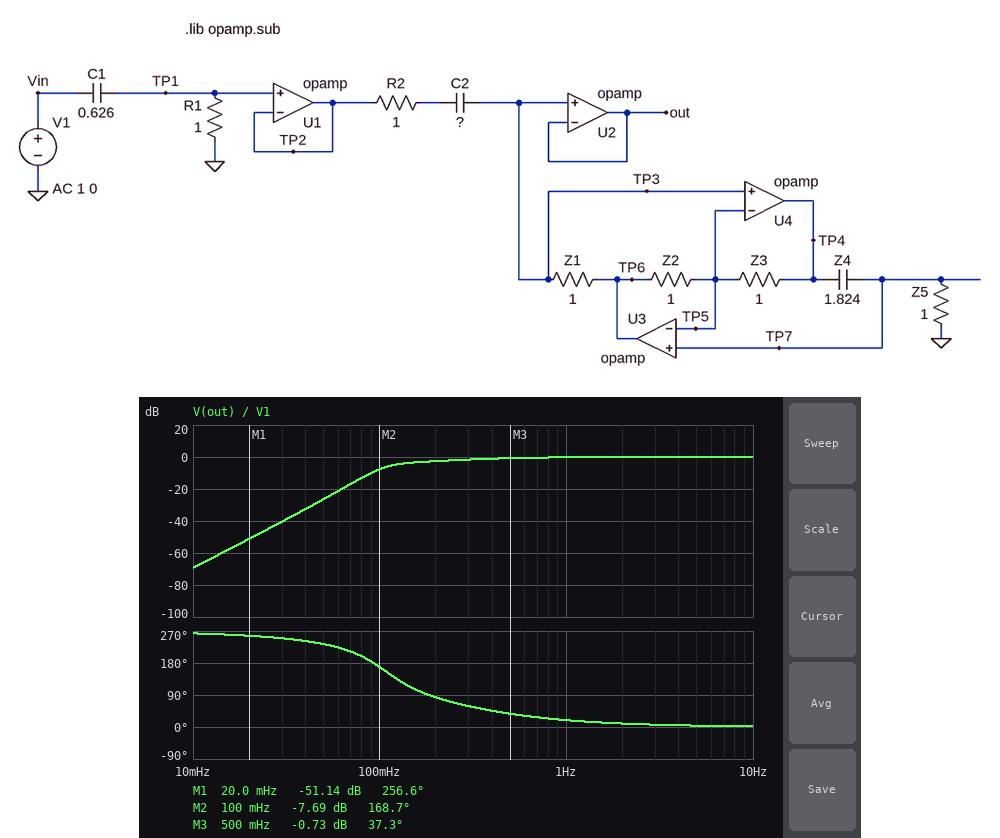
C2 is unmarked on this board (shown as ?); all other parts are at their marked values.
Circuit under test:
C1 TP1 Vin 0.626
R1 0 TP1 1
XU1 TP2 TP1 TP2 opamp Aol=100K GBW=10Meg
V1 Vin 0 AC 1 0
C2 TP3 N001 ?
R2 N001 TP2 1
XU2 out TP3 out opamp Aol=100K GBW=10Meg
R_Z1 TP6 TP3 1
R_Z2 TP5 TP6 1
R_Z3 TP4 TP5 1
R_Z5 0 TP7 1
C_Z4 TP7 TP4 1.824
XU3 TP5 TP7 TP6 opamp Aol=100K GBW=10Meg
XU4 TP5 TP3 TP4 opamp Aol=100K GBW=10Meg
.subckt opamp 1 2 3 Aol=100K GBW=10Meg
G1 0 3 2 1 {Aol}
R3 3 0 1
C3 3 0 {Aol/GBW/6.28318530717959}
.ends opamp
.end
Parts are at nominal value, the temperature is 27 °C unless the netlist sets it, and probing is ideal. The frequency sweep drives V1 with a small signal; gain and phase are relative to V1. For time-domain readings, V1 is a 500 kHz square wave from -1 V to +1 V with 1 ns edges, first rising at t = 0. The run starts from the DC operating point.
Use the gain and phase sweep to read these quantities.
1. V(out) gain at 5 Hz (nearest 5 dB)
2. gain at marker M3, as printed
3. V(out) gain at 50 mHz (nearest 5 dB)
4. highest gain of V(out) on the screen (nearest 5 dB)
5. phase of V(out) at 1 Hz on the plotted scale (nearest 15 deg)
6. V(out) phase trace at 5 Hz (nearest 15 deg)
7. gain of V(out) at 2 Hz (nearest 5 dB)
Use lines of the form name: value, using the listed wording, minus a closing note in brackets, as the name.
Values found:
V(out) gain at 5 Hz: 0 dB
gain at marker M3, as printed: -0.73 dB
V(out) gain at 50 mHz: -25 dB
highest gain of V(out) on the screen: 0 dB
phase of V(out) at 1 Hz on the plotted scale: 15 deg
V(out) phase trace at 5 Hz: 0 deg
gain of V(out) at 2 Hz: 0 dB
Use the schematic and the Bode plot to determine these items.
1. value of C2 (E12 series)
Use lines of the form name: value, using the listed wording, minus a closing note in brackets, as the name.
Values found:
value of C2: 1.2 F
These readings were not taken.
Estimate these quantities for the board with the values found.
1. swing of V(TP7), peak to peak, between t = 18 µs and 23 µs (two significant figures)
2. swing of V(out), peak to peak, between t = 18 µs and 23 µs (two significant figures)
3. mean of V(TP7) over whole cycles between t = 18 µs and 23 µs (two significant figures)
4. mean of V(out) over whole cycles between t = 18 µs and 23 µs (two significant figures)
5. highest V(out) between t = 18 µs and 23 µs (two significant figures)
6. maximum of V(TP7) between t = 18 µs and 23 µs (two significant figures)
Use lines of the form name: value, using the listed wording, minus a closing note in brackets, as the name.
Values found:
swing of V(TP7), peak to peak, between t = 18 µs and 23 µs: 2.0 V
swing of V(out), peak to peak, between t = 18 µs and 23 µs: 2.0 V
mean of V(TP7) over whole cycles between t = 18 µs and 23 µs: 1.0 V
mean of V(out) over whole cycles between t = 18 µs and 23 µs: 1.0 V
highest V(out) between t = 18 µs and 23 µs: 2.0 V
maximum of V(TP7) between t = 18 µs and 23 µs: 2.0 V
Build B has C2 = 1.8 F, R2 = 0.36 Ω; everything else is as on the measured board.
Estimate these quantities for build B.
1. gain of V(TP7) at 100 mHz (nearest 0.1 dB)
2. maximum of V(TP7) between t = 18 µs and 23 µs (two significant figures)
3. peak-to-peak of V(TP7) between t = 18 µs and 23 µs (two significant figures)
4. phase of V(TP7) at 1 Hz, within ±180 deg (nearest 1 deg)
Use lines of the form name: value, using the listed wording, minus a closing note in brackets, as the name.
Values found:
gain of V(TP7) at 100 mHz: -0.5 dB
maximum of V(TP7) between t = 18 µs and 23 µs: 2.1 V
peak-to-peak of V(TP7) between t = 18 µs and 23 µs: 2.2 V
phase of V(TP7) at 1 Hz, within ±180 deg: 16 deg
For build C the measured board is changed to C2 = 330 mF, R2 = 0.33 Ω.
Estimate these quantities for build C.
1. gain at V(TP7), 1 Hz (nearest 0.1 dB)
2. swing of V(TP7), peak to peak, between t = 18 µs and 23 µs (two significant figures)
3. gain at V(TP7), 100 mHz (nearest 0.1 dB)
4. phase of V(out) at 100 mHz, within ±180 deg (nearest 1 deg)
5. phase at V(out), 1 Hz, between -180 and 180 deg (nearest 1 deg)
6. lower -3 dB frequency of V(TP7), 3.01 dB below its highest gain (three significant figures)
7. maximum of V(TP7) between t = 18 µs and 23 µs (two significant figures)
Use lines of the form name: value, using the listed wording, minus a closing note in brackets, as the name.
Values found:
gain at V(TP7), 1 Hz: 0.1 dB
swing of V(TP7), peak to peak, between t = 18 µs and 23 µs: 2.2 V
gain at V(TP7), 100 mHz: -18.9 dB
phase of V(out) at 100 mHz, within ±180 deg: -117 deg
phase at V(out), 1 Hz, between -180 and 180 deg: 16 deg
lower -3 dB frequency of V(TP7), 3.01 dB below its highest gain: 194 mHz
maximum of V(TP7) between t = 18 µs and 23 µs: 2.1 V
